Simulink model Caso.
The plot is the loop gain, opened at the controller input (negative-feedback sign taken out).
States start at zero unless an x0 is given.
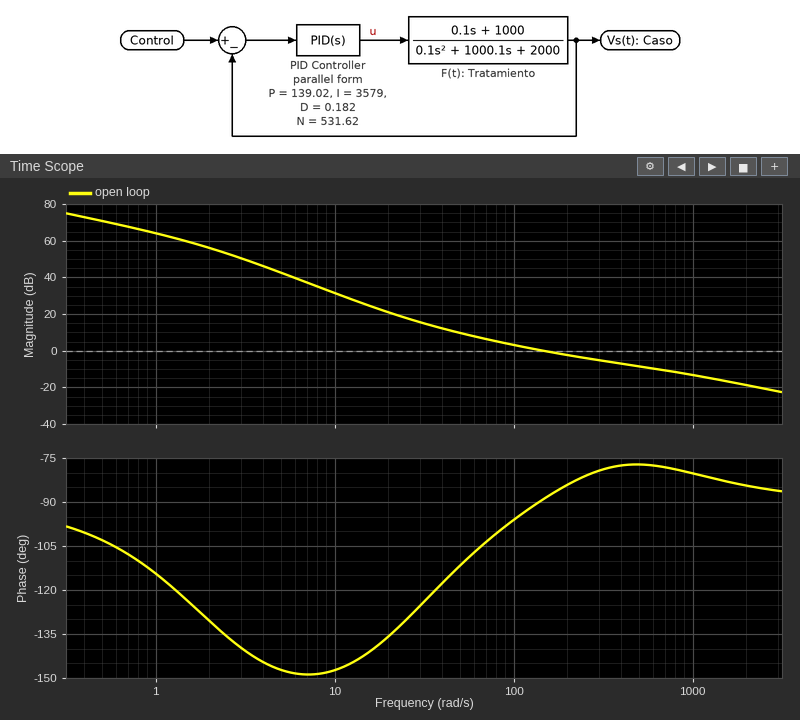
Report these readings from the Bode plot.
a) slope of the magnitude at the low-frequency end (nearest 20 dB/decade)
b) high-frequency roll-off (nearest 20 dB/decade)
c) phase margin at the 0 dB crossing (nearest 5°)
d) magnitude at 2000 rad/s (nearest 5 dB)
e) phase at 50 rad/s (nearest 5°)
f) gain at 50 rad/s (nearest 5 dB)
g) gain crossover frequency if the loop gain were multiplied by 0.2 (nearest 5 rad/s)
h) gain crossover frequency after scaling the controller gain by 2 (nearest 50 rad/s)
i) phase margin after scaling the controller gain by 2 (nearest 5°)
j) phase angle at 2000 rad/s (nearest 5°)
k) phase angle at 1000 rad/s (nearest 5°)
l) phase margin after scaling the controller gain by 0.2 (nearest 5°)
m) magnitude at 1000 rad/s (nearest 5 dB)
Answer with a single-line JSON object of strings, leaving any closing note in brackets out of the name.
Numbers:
{"slope of the magnitude at the low-frequency end": "-20 dB/decade", "high-frequency roll-off": "-20 dB/decade", "phase margin at the 0 dB crossing": "90°", "magnitude at 2000 rad/s": "-20 dB", "phase at 50 rad/s": "-110°", "gain at 50 rad/s": "10 dB", "gain crossover frequency if the loop gain were multiplied by 0.2": "35 rad/s", "gain crossover frequency after scaling the controller gain by 2": "350 rad/s", "phase margin after scaling the controller gain by 2": "100°", "phase angle at 2000 rad/s": "-85°", "phase angle at 1000 rad/s": "-80°", "phase margin after scaling the controller gain by 0.2": "60°", "magnitude at 1000 rad/s": "-15 dB"}
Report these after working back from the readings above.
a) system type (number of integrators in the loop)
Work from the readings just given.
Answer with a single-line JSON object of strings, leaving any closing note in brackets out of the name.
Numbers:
{"system type": "1"}
